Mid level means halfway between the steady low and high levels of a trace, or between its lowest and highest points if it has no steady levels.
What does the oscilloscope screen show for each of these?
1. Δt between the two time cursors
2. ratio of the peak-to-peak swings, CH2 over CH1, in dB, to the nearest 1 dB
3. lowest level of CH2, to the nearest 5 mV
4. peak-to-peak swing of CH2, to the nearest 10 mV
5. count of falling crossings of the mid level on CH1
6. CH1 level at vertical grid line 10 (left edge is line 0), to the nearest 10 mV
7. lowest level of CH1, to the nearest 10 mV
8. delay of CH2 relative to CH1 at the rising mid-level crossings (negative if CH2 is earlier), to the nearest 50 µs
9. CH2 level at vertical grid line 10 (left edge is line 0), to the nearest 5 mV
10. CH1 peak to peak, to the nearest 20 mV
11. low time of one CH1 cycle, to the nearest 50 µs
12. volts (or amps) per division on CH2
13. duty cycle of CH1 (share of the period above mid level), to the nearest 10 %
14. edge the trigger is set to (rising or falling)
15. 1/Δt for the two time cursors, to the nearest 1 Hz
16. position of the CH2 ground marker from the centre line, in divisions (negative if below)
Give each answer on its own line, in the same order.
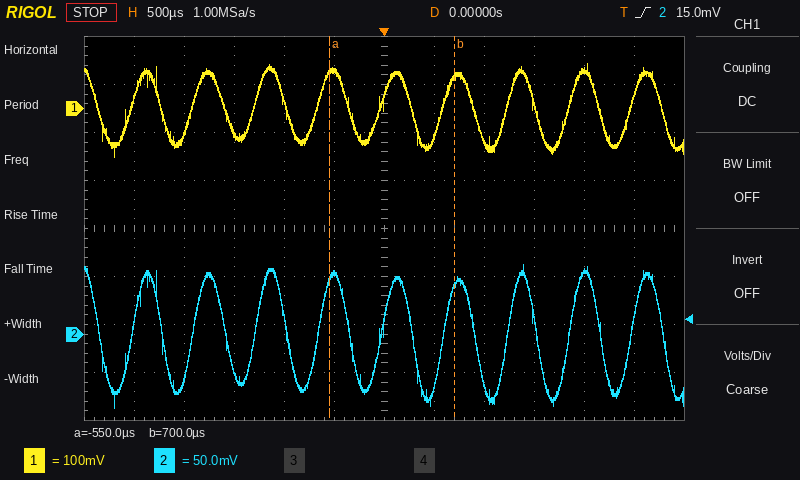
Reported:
1.25 ms
-2 dB
-75 mV
150 mV
10
80 mV
-100 mV
0 µs
65 mV
200 mV
300 µs
50 mV
50 %
rising
800 Hz
-2.2 div
